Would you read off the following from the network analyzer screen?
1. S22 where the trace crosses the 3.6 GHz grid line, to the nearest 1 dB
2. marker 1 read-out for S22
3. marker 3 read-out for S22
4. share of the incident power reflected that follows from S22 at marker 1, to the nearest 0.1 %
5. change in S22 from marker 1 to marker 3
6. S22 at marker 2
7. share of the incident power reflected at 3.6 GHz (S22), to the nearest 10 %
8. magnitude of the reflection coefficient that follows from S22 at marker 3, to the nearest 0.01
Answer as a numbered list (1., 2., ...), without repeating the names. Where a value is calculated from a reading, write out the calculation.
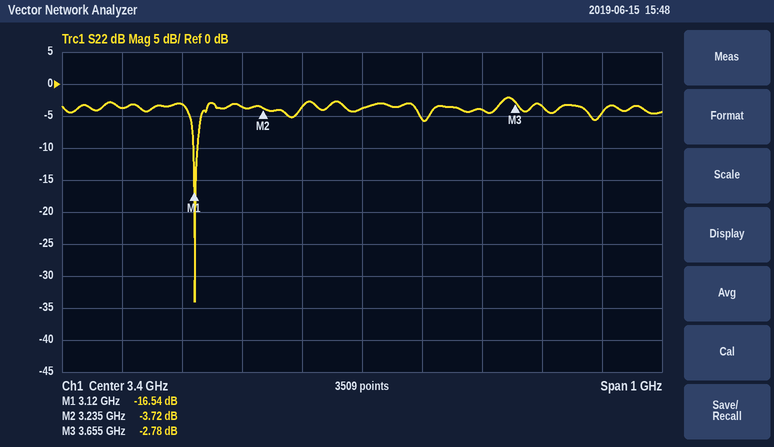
1. -4 dB
2. -16.54 dB
3. -2.78 dB
4. 10^(-16.54/10) ≈ 2.2 %
5. -2.78 − (-16.54) = 13.76 dB
6. -3.72 dB
7. 10^(-4/10) ≈ 40 %
8. 10^(-2.78/20) ≈ 0.73
